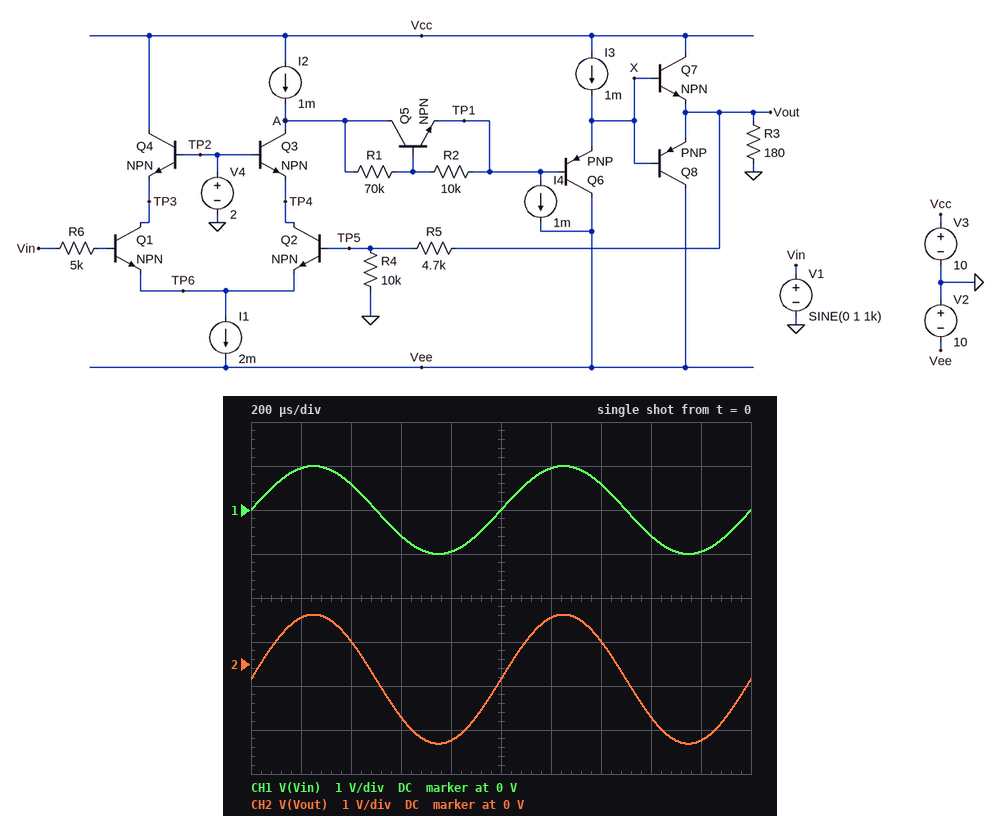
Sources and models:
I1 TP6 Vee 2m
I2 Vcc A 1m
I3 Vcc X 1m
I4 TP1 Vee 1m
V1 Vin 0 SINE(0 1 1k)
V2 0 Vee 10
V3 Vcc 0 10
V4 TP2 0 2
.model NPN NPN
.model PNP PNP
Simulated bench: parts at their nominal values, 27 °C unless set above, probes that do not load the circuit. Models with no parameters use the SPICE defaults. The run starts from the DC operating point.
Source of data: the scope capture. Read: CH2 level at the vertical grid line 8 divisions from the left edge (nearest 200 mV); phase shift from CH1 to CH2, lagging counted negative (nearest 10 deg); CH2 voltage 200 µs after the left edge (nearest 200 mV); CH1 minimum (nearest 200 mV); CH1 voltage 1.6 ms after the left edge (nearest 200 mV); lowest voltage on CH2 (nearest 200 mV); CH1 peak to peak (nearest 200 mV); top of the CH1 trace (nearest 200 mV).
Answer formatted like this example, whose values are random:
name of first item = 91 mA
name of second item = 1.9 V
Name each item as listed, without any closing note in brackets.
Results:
CH2 level at the vertical grid line 8 divisions from the left edge = -1.2 V
phase shift from CH1 to CH2, lagging counted negative = 0 deg
CH2 voltage 200 µs after the left edge = 1.0 V
CH1 minimum = -1.0 V
CH1 voltage 1.6 ms after the left edge = -600 mV
lowest voltage on CH2 = -1.8 V
CH1 peak to peak = 2.0 V
top of the CH1 trace = 1.0 V
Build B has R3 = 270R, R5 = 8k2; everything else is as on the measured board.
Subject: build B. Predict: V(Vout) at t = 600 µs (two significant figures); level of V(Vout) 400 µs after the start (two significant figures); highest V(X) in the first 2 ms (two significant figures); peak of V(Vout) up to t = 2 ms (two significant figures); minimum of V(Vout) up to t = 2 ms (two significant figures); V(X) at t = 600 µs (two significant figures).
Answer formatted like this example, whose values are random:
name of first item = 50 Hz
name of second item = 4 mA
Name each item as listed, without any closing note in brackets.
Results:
V(Vout) at t = 600 µs = -1.5 V
level of V(Vout) 400 µs after the start = 640 mV
highest V(X) in the first 2 ms = 2.2 V
peak of V(Vout) up to t = 2 ms = 1.4 V
minimum of V(Vout) up to t = 2 ms = -2.2 V
V(X) at t = 600 µs = -2.3 V
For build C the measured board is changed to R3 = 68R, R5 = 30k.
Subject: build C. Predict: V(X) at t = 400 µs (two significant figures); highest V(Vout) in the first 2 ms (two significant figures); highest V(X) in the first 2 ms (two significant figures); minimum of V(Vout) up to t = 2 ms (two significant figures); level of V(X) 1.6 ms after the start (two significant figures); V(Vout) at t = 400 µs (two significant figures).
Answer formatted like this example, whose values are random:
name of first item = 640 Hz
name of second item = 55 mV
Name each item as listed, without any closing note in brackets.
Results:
V(X) at t = 400 µs = 2.2 V
highest V(Vout) in the first 2 ms = 3.0 V
highest V(X) in the first 2 ms = 3.9 V
minimum of V(Vout) up to t = 2 ms = -3.9 V
level of V(X) 1.6 ms after the start = -4.1 V
V(Vout) at t = 400 µs = 1.4 V
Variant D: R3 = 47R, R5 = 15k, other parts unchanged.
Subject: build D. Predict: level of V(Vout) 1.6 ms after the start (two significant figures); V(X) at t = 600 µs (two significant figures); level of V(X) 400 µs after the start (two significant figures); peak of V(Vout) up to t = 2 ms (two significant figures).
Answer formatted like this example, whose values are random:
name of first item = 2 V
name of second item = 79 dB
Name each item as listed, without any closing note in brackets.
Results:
level of V(Vout) 1.6 ms after the start = -2.0 V
V(X) at t = 600 µs = -2.9 V
level of V(X) 400 µs after the start = 1.7 V
peak of V(Vout) up to t = 2 ms = 1.9 V
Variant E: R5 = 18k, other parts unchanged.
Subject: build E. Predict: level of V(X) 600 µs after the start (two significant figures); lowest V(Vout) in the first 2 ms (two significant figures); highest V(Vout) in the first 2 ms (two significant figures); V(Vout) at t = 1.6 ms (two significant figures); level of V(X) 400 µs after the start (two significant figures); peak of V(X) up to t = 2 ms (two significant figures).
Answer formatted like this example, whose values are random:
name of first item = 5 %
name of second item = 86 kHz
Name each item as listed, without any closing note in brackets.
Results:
level of V(X) 600 µs after the start = -3.1 V
lowest V(Vout) in the first 2 ms = -3.4 V
highest V(Vout) in the first 2 ms = 2.1 V
V(Vout) at t = 1.6 ms = -2.3 V
level of V(X) 400 µs after the start = 1.8 V
peak of V(X) up to t = 2 ms = 3.0 V
